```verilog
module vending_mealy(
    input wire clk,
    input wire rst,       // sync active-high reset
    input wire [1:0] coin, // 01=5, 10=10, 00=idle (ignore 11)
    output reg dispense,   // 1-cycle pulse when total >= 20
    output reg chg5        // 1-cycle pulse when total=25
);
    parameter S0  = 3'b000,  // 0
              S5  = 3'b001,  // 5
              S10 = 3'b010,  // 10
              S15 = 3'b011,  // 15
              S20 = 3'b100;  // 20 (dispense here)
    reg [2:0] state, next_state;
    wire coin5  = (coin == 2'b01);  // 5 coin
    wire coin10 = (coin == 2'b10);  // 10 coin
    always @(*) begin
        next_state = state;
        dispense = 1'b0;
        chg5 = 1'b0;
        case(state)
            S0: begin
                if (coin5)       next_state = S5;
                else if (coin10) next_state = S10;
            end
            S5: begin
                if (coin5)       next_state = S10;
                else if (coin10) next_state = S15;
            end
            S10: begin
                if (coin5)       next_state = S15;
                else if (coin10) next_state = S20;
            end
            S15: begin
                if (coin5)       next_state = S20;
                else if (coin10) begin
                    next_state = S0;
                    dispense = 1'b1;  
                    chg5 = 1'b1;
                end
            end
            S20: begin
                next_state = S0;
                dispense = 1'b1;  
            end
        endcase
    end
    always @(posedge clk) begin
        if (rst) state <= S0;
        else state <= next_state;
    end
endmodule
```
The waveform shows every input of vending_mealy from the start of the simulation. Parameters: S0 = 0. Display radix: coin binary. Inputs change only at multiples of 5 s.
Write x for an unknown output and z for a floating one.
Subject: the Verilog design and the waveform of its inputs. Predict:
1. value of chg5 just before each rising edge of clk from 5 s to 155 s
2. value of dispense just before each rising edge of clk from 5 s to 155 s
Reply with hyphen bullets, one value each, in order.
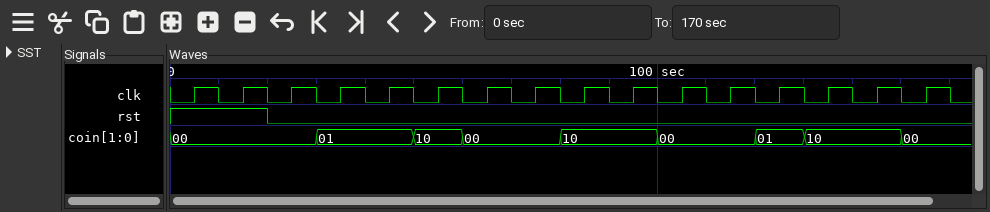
- 0 0 0 0 0 0 0 0 0 0 0 0 0 0 1 0
- 0 0 0 0 0 0 1 0 0 0 1 0 0 0 1 0
